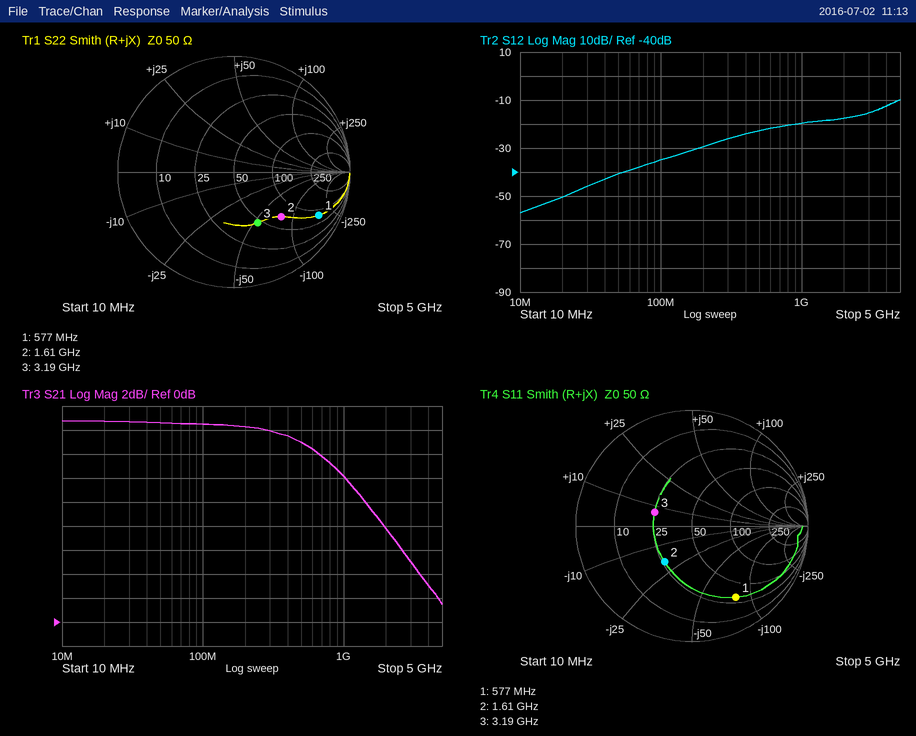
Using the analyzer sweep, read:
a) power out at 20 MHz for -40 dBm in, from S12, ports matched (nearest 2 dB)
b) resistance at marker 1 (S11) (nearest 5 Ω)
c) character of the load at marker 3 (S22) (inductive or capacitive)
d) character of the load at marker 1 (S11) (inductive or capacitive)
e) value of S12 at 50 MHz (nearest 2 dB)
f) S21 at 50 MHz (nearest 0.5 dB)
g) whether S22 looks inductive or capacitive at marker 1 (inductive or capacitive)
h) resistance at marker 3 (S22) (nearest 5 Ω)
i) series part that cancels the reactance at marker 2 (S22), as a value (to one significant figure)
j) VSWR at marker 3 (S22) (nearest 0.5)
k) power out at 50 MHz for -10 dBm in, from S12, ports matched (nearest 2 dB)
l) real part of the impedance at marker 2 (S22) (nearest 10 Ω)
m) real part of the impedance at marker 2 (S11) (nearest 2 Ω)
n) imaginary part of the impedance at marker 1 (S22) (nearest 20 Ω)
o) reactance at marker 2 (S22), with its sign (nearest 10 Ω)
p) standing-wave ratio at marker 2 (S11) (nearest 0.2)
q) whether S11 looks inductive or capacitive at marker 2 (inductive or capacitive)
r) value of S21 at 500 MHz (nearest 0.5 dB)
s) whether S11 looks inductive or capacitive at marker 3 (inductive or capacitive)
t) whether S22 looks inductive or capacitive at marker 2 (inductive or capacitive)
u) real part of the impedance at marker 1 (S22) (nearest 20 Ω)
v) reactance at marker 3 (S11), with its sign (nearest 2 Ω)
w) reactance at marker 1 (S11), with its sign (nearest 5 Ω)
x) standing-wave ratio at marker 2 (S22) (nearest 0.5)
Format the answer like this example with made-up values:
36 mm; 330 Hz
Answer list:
-90 dBm; 30 Ω; capacitive; capacitive; -40 dB; 16.5 dB; capacitive; 45 Ω; 8 nH; 3.0; -50 dBm; 70 Ω; 26 Ω; -180 Ω; -80 Ω; 2.2; capacitive; 15.0 dB; inductive; capacitive; 80 Ω; +6 Ω; -80 Ω; 3.5
